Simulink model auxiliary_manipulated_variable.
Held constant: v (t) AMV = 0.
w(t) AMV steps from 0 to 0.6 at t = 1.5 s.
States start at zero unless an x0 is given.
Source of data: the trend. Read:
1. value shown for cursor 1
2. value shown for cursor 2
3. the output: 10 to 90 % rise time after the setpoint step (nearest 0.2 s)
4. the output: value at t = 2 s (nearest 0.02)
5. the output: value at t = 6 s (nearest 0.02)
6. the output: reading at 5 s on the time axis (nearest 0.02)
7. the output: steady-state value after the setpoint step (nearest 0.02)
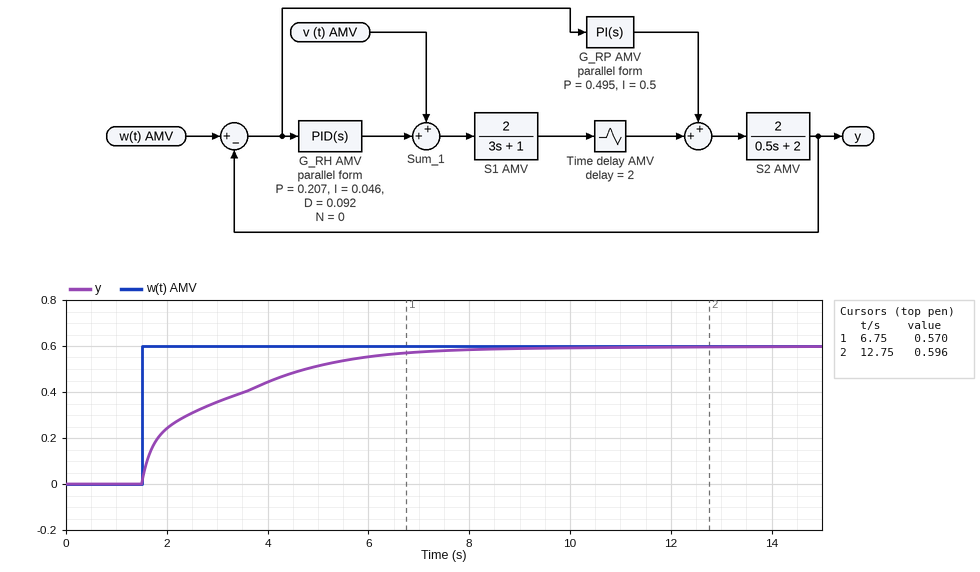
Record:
0.570
0.596
4.0 s
0.24
0.56
0.52
0.60
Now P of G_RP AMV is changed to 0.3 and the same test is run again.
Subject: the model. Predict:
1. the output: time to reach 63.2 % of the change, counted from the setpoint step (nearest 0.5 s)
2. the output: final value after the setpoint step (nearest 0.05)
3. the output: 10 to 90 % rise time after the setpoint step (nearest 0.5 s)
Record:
2.0 s
0.60
3.5 s
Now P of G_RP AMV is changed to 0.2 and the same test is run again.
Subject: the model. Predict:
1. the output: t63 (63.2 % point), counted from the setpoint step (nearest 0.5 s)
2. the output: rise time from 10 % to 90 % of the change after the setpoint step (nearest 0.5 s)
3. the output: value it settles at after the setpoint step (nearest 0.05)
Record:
2.0 s
3.5 s
0.60
